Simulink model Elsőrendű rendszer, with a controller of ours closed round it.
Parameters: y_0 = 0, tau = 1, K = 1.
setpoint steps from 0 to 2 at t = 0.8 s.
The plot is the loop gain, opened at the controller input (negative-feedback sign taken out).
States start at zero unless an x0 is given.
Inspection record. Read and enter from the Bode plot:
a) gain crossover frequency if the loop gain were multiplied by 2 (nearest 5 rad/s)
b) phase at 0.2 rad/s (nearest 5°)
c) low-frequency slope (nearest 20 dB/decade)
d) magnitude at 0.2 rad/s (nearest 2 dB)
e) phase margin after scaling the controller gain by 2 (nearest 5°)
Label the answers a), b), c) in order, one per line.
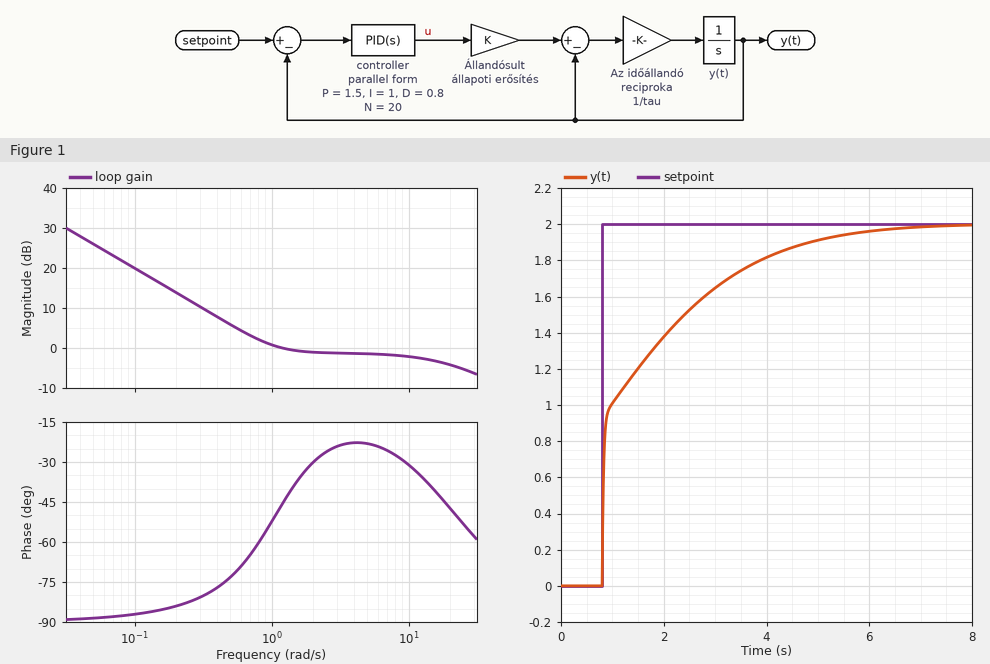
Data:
a) 30 rad/s
b) -85°
c) -20 dB/decade
d) 14 dB
e) 125°
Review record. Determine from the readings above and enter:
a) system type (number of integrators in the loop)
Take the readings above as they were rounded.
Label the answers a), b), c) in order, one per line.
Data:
a) 1
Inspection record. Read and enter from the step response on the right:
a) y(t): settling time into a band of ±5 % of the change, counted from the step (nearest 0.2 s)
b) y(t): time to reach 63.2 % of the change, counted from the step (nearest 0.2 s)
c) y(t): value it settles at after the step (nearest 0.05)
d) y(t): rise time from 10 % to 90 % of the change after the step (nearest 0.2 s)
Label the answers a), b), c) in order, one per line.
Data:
a) 4.0 s
b) 0.8 s
c) 2.00
d) 3.0 s
